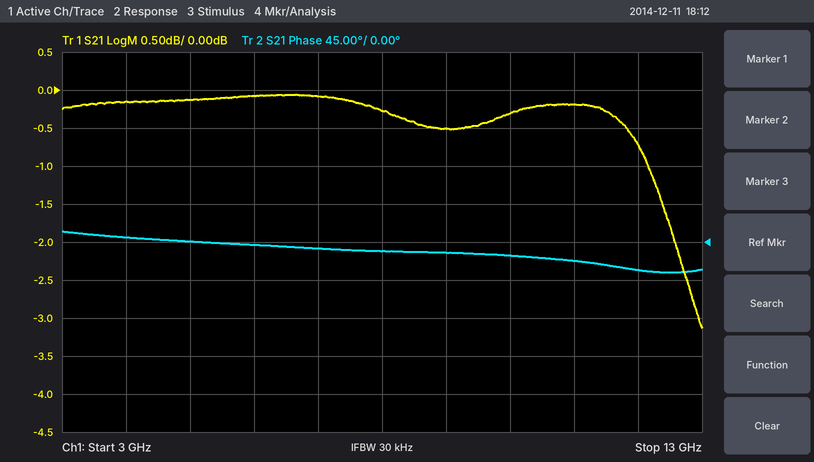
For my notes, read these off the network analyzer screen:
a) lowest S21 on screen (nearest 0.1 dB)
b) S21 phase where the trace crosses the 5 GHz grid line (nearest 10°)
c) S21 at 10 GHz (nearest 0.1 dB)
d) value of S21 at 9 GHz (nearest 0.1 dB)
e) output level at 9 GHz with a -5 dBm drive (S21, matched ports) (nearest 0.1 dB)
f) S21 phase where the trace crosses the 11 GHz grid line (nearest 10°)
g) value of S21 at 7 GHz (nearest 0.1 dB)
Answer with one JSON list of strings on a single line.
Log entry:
["-3.1 dB", "0°", "-0.3 dB", "-0.5 dB", "-5.5 dBm", "-20°", "-0.1 dB"]
